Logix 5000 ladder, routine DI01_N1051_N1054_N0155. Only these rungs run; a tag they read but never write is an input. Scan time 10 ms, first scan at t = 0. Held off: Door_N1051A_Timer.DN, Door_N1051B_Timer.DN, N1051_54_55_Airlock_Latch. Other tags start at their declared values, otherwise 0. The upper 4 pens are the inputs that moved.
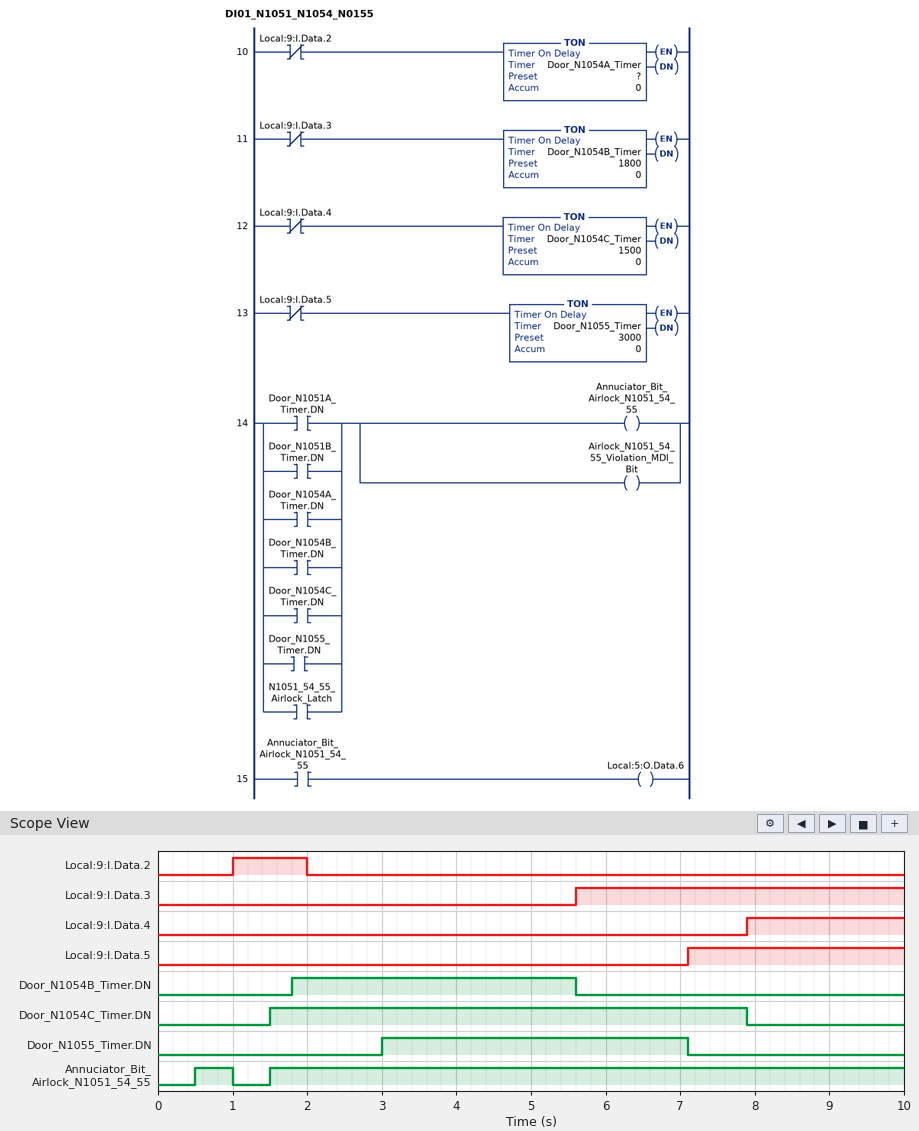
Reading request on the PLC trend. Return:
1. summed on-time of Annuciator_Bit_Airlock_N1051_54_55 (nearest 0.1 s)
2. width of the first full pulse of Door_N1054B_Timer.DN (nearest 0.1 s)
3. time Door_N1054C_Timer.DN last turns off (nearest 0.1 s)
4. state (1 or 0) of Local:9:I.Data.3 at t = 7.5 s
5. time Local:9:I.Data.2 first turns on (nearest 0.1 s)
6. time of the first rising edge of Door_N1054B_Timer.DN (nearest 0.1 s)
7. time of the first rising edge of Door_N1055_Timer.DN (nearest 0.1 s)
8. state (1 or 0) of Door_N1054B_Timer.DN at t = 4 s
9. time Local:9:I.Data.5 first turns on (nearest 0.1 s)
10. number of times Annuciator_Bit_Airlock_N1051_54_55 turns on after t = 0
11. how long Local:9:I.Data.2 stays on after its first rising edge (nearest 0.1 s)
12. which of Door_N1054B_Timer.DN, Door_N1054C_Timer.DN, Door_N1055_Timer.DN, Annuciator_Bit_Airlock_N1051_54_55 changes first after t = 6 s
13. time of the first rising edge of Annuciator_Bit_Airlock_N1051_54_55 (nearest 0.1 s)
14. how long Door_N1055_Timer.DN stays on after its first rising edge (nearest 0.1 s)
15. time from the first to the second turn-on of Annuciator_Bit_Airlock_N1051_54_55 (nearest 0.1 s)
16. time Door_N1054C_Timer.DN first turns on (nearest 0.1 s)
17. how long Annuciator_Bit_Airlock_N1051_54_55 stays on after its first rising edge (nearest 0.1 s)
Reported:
9.0 s
3.8 s
7.9 s
1
1.0 s
1.8 s
3.0 s
1
7.1 s
2
1.0 s
Door_N1055_Timer.DN
0.5 s
4.1 s
1.0 s
1.5 s
0.5 s
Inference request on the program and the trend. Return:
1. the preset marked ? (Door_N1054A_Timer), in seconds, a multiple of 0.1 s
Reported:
0.5 s
